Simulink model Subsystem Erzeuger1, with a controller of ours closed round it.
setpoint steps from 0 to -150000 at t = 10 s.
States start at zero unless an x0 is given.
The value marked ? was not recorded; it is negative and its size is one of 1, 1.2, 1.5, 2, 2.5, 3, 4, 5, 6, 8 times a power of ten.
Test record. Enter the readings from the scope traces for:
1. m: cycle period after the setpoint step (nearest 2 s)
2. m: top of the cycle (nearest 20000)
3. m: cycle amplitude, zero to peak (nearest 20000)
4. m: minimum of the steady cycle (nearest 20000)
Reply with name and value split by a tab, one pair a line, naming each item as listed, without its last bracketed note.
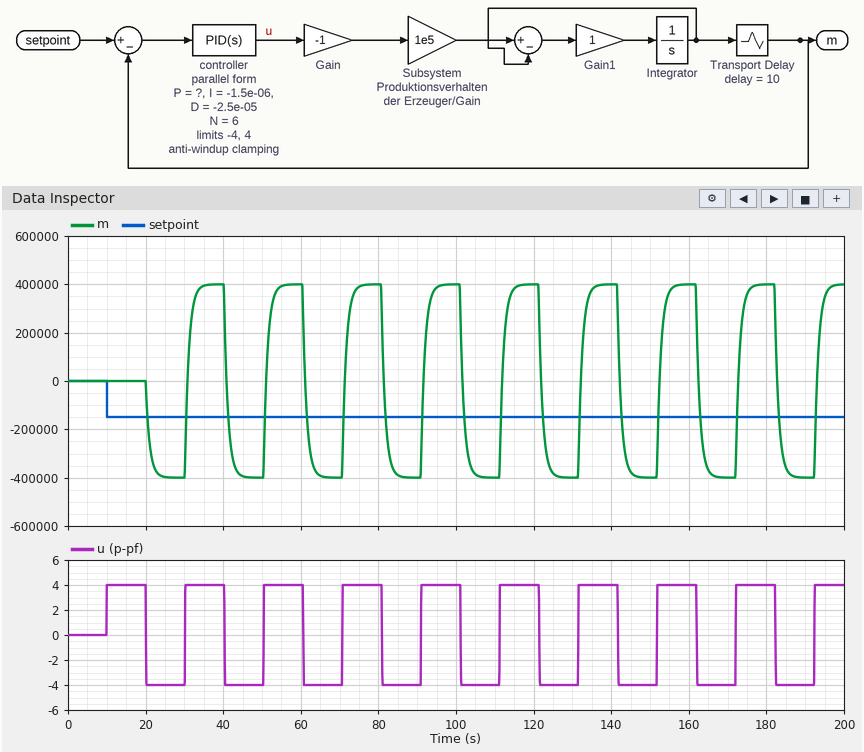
m: cycle period after the setpoint step	20 s
m: top of the cycle	400000
m: cycle amplitude, zero to peak	400000
m: minimum of the steady cycle	-400000
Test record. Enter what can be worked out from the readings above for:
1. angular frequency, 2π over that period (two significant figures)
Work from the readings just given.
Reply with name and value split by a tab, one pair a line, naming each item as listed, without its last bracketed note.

angular frequency, 2π over that period	0.31 rad/s
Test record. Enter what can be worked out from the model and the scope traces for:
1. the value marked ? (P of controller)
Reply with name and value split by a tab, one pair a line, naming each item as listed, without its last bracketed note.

the value marked ?	-3e-05
